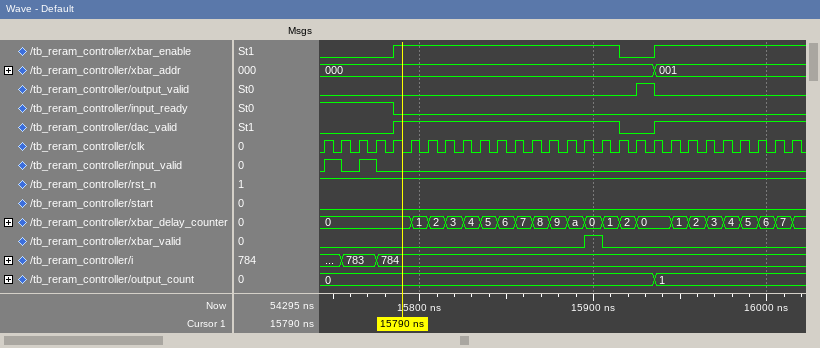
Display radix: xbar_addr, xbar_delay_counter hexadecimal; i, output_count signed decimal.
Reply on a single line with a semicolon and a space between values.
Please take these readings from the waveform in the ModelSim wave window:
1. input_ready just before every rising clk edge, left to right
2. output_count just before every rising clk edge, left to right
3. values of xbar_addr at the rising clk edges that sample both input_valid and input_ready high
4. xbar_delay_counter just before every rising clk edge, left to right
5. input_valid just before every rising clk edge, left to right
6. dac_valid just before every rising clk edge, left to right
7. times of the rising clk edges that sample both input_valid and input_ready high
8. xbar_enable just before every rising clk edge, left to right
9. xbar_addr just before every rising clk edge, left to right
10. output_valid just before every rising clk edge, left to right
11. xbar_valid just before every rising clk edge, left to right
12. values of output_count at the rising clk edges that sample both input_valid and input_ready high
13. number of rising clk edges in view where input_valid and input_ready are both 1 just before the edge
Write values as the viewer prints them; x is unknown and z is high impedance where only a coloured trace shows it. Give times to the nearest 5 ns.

1 1 1 1 1 0 0 0 0 0 0 0 0 0 0 0 0 0 0 0 0 0 0 0 0 0 0 0; 0, 0, 0, 0, 0, 0, 0, 0, 0, 0, 0, 0, 0, 0, 0, 0, 0, 0, 0, 0, 1, 1, 1, 1, 1, 1, 1, 1; 000, 000; 0, 0, 0, 0, 0, 0, 1, 2, 3, 4, 5, 6, 7, 8, 9, a, 0, 1, 2, 0, 0, 1, 2, 3, 4, 5, 6, 7; 0 1 0 1 0 0 0 0 0 0 0 0 0 0 0 0 0 0 0 0 0 0 0 0 0 0 0 0; 0 0 0 0 0 1 1 1 1 1 1 1 1 1 1 1 1 1 0 0 1 1 1 1 1 1 1 1; 15755 ns, 15775 ns; 0 0 0 0 0 1 1 1 1 1 1 1 1 1 1 1 1 1 0 0 1 1 1 1 1 1 1 1; 000, 000, 000, 000, 000, 000, 000, 000, 000, 000, 000, 000, 000, 000, 000, 000, 000, 000, 000, 000, 001, 001, 001, 001, 001, 001, 001, 001; 0 0 0 0 0 0 0 0 0 0 0 0 0 0 0 0 0 0 0 1 0 0 0 0 0 0 0 0; 0 0 0 0 0 0 0 0 0 0 0 0 0 0 0 0 1 0 0 0 0 0 0 0 0 0 0 0; 0, 0; 2
